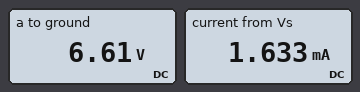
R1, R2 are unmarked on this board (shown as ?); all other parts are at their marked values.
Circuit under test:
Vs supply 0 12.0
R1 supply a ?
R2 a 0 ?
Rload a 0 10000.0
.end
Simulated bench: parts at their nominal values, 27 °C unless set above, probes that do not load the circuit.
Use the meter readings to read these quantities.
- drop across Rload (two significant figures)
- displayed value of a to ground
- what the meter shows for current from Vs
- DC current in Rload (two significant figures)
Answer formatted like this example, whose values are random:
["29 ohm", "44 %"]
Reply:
["6.6 V", "6.61 V", "1.633 mA", "660 µA"]
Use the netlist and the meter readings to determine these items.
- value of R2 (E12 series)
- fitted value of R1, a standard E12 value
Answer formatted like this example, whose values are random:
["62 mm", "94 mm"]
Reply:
["6.8 kΩ", "3.3 kΩ"]
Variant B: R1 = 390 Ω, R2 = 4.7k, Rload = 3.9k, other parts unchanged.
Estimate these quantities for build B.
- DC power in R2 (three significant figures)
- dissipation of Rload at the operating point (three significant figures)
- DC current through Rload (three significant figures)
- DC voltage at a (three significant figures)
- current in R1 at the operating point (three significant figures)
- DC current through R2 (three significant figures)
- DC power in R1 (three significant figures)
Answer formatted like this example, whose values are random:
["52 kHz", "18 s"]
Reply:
["21.9 mW", "26.4 mW", "2.60 mA", "10.1 V", "4.76 mA", "2.16 mA", "8.83 mW"]
